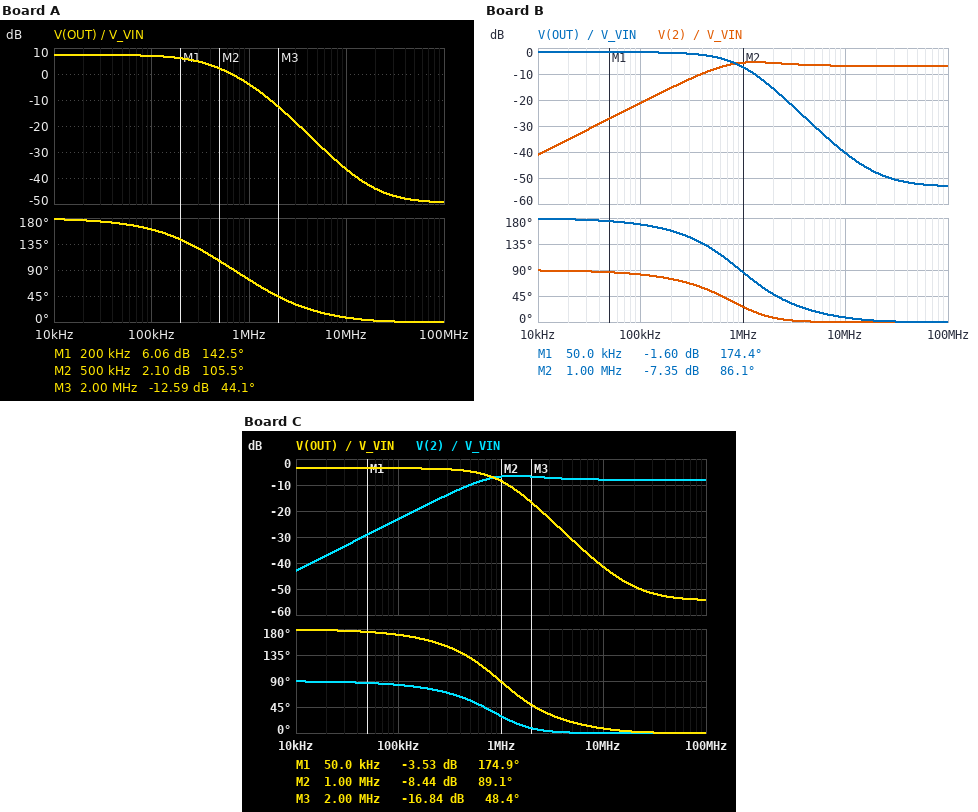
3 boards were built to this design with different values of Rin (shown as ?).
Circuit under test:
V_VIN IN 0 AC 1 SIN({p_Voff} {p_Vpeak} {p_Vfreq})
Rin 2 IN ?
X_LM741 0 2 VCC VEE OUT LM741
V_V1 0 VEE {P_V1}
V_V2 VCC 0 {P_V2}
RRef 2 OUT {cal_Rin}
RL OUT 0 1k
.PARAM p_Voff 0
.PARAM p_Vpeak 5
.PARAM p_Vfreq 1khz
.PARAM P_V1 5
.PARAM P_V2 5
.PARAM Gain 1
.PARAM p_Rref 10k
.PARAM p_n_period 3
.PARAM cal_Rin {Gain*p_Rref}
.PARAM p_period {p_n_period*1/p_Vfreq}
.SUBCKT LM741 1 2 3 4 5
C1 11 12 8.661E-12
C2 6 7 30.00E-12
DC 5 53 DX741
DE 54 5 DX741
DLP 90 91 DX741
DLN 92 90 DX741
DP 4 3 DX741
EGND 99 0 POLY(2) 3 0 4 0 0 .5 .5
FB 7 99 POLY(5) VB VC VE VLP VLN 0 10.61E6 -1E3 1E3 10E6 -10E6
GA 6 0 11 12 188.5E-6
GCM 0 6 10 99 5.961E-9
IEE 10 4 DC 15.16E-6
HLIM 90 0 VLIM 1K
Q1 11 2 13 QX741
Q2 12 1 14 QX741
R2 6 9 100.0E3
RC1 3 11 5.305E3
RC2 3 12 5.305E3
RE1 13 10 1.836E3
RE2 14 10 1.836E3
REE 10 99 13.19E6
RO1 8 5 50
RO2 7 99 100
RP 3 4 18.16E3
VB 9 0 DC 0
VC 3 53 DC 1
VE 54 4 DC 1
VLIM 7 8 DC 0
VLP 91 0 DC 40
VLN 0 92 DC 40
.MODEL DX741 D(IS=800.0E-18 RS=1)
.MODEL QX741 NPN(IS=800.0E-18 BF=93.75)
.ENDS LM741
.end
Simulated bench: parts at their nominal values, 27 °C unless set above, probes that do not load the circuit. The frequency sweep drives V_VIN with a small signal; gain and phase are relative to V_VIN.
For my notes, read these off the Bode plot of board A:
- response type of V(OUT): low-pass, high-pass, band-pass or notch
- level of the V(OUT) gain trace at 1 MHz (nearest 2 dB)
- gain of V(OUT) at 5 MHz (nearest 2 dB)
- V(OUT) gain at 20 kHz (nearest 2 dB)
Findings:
low-pass
-4 dB
-26 dB
8 dB
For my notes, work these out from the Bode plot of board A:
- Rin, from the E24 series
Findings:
4.3 kΩ
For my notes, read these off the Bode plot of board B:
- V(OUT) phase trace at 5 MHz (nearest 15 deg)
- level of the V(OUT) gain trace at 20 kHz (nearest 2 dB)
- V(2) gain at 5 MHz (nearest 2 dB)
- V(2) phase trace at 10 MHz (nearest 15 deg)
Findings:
15 deg
-2 dB
-6 dB
0 deg
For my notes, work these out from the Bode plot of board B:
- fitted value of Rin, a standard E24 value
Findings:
12 kΩ
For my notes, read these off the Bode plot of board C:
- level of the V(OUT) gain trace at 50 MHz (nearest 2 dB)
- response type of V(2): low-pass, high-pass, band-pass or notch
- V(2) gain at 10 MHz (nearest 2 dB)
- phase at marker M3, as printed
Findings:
-54 dB
high-pass
-8 dB
48.4 deg
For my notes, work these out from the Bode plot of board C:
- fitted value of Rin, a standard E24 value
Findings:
15 kΩ
